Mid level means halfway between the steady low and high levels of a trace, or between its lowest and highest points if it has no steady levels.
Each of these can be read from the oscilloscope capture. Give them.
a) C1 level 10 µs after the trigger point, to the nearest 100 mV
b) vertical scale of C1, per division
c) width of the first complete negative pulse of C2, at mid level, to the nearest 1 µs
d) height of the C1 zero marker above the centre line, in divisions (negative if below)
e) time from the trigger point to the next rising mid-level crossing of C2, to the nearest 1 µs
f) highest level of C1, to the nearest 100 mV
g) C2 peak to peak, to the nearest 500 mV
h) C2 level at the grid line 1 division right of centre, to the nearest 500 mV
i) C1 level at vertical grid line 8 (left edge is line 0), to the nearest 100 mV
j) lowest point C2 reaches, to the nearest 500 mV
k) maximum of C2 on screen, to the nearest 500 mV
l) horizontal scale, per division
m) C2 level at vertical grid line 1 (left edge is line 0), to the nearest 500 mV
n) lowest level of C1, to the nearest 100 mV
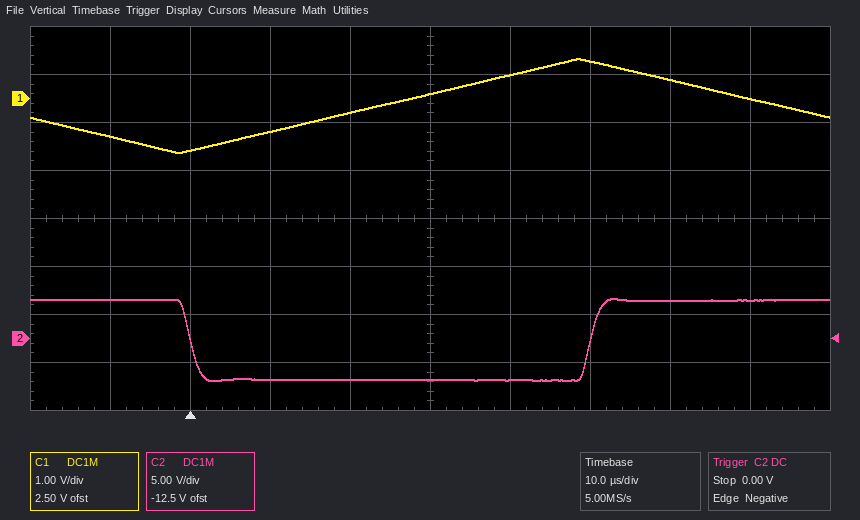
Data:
-700 mV
1 V
50 µs
+2.5 div
50 µs
800 mV
8.5 V
-4.5 V
400 mV
-4.5 V
4.0 V
10 µs
4.0 V
-1.1 V
